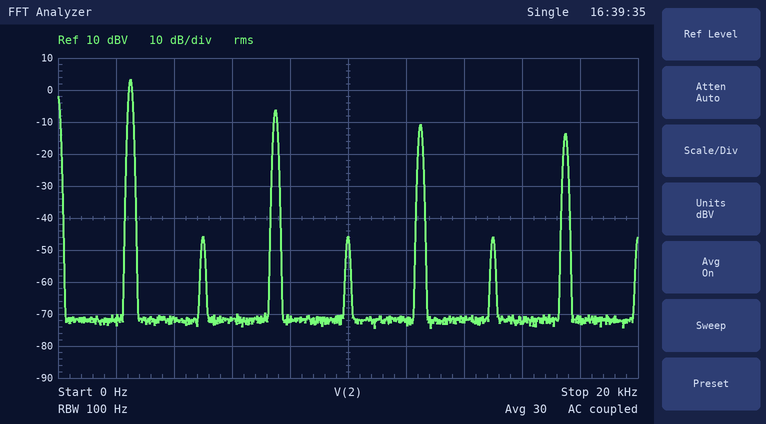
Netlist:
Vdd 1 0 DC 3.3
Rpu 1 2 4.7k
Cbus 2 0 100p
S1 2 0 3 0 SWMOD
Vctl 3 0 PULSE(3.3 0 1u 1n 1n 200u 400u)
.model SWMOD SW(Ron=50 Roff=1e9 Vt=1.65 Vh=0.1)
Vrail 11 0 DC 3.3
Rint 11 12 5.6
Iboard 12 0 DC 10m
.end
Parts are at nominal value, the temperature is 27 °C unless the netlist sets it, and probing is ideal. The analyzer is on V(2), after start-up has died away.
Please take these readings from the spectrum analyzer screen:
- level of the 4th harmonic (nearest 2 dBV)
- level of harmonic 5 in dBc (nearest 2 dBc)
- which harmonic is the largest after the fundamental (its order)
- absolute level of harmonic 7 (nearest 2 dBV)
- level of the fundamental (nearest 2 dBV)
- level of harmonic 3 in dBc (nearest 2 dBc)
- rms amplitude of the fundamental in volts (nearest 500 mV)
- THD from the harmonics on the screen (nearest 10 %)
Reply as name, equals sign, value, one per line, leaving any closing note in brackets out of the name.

level of the 4th harmonic = -46 dBV
level of harmonic 5 in dBc = -14 dBc
which harmonic is the largest after the fundamental = 3
absolute level of harmonic 7 = -14 dBV
level of the fundamental = 4 dBV
level of harmonic 3 in dBc = -10 dBc
rms amplitude of the fundamental in volts = 1.5 V
THD from the harmonics on the screen = 40 %
